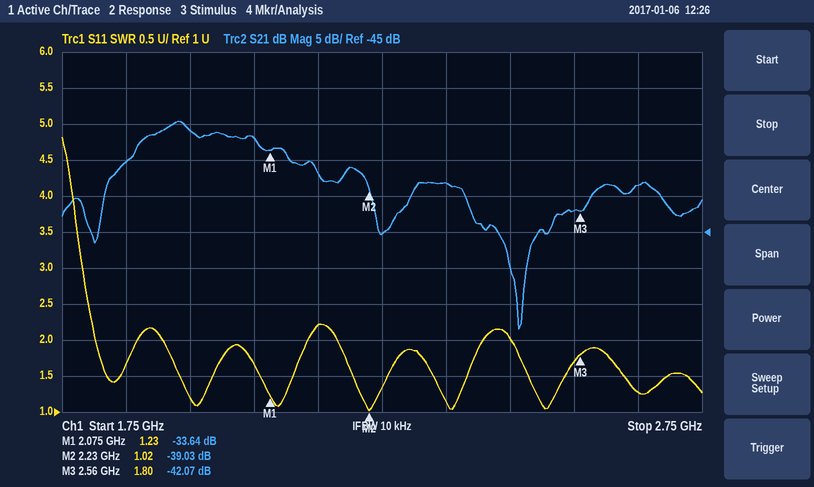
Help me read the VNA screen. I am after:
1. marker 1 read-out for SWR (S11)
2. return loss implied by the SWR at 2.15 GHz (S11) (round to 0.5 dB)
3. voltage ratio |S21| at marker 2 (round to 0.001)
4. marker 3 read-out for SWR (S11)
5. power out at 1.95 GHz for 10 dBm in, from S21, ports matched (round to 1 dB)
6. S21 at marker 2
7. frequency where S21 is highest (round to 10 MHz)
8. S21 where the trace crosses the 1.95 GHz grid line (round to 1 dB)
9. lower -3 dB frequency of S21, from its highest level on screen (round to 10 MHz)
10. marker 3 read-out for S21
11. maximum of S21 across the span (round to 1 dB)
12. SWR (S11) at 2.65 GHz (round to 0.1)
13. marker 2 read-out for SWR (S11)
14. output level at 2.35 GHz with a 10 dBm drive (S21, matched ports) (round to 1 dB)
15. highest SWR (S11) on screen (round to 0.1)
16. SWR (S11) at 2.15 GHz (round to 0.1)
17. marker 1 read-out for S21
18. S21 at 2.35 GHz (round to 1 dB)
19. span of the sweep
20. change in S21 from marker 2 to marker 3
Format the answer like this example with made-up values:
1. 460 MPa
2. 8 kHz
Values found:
1. 1.23
2. 8.5 dB
3. 0.011
4. 1.80
5. -21 dBm
6. -39.03 dB
7. 1.93 GHz
8. -31 dB
9. 1.87 GHz
10. -42.07 dB
11. -30 dB
12. 1.3
13. 1.02
14. -28 dBm
15. 4.8
16. 2.2
17. -33.64 dB
18. -38 dB
19. 1 GHz
20. -3.04 dB
